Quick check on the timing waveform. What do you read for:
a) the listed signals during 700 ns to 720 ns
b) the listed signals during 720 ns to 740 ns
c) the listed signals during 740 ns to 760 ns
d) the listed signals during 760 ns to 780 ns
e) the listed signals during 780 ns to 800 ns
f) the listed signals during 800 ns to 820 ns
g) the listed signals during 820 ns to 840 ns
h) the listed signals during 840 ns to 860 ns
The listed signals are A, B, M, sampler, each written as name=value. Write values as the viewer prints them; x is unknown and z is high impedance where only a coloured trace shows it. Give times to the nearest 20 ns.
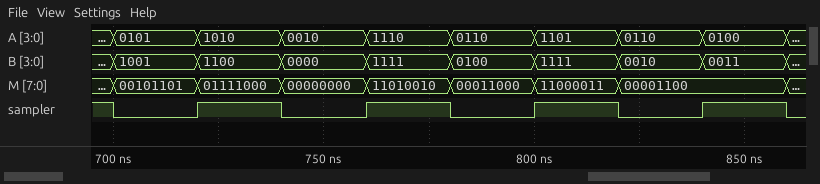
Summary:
A=0101, B=1001, M=00101101, sampler=0
A=1010, B=1100, M=01111000, sampler=1
A=0010, B=0000, M=00000000, sampler=0
A=1110, B=1111, M=11010010, sampler=1
A=0110, B=0100, M=00011000, sampler=0
A=1101, B=1111, M=11000011, sampler=1
A=0110, B=0010, M=00001100, sampler=0
A=0100, B=0011, M=00001100, sampler=1
